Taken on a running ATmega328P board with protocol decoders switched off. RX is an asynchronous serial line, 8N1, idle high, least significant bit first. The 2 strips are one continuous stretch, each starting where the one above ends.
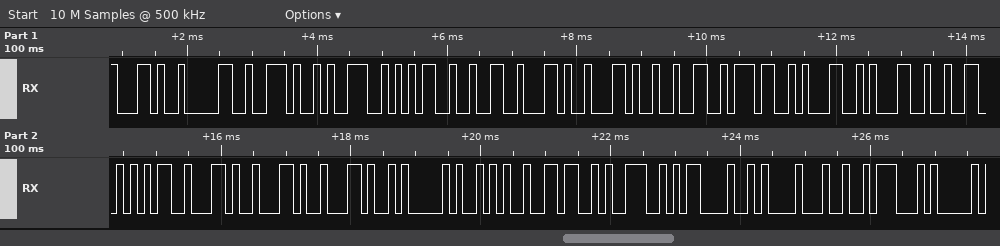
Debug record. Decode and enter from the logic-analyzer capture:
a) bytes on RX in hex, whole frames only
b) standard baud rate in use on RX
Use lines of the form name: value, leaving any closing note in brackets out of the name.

bytes on RX in hex, whole frames only: 0x2C 0x30 0x2E 0x39 0x35 0x32 0x2C 0x2C 0x32 0x37 0x31 0x31 0x32 0x35 0x2C 0x2C 0x2C 0x41 0x2A 0x36 0x39 0x0D 0x0A 0x24 0x47
standard baud rate in use on RX: 9600 baud
